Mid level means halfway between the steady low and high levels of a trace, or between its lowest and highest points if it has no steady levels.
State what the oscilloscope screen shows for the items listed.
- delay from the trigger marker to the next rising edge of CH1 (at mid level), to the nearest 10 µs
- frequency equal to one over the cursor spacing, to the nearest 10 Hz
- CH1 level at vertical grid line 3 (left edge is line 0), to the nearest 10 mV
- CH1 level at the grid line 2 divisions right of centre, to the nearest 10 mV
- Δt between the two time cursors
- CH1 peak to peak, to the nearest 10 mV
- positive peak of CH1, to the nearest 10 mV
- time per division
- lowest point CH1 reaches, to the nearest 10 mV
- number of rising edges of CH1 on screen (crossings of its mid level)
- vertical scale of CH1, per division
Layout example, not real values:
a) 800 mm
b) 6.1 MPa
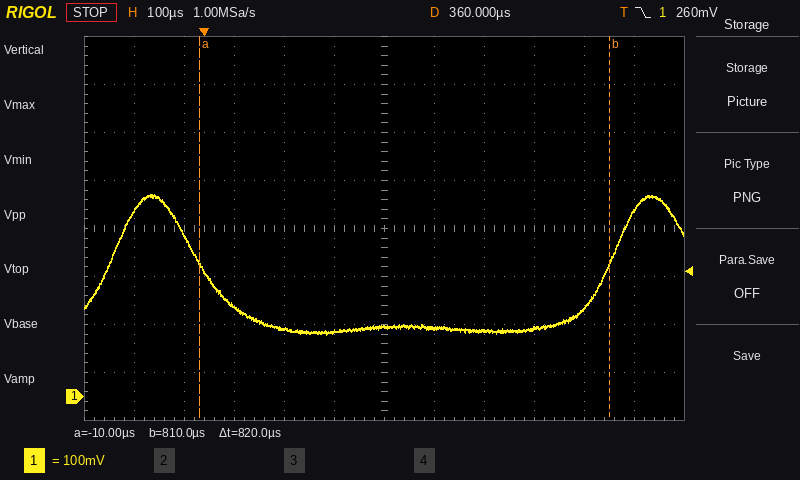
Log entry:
a) 810 µs
b) 1.22 kHz
c) 190 mV
d) 140 mV
e) 820 µs
f) 290 mV
g) 420 mV
h) 100 µs
i) 130 mV
j) 2
k) 100 mV
